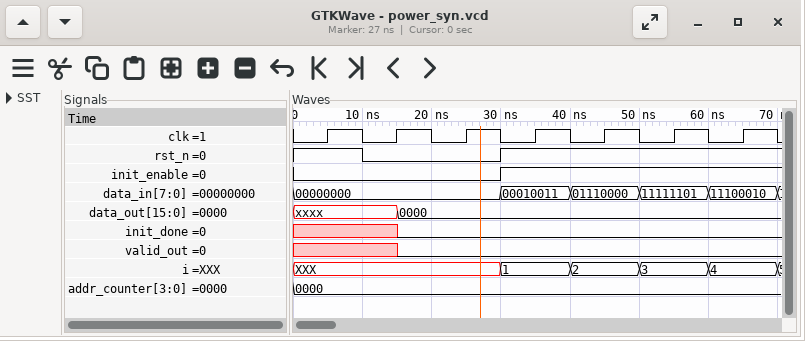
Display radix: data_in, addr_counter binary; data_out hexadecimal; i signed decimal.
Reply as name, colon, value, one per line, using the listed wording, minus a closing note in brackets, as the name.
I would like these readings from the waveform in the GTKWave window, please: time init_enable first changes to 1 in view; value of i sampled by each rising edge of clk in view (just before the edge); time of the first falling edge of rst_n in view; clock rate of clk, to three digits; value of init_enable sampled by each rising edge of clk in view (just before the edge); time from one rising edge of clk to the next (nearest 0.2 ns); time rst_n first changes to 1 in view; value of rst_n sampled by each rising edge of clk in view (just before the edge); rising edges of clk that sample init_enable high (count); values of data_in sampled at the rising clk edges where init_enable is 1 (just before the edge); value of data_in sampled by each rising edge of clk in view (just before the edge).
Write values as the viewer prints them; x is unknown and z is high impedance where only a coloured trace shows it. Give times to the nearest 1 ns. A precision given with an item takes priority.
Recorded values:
time init_enable first changes to 1 in view: 30 ns
value of i sampled by each rising edge of clk in view: XXX, XXX, XXX, 1, 2, 3, 4
time of the first falling edge of rst_n in view: 10 ns
clock rate of clk, to three digits: 100 MHz
value of init_enable sampled by each rising edge of clk in view: 0 0 0 1 1 1 1
time from one rising edge of clk to the next: 10 ns
time rst_n first changes to 1 in view: 30 ns
value of rst_n sampled by each rising edge of clk in view: 1 0 0 1 1 1 1
rising edges of clk that sample init_enable high: 4
values of data_in sampled at the rising clk edges where init_enable is 1: 00010011, 01110000, 11111101, 11100010
value of data_in sampled by each rising edge of clk in view: 00000000, 00000000, 00000000, 00010011, 01110000, 11111101, 11100010
